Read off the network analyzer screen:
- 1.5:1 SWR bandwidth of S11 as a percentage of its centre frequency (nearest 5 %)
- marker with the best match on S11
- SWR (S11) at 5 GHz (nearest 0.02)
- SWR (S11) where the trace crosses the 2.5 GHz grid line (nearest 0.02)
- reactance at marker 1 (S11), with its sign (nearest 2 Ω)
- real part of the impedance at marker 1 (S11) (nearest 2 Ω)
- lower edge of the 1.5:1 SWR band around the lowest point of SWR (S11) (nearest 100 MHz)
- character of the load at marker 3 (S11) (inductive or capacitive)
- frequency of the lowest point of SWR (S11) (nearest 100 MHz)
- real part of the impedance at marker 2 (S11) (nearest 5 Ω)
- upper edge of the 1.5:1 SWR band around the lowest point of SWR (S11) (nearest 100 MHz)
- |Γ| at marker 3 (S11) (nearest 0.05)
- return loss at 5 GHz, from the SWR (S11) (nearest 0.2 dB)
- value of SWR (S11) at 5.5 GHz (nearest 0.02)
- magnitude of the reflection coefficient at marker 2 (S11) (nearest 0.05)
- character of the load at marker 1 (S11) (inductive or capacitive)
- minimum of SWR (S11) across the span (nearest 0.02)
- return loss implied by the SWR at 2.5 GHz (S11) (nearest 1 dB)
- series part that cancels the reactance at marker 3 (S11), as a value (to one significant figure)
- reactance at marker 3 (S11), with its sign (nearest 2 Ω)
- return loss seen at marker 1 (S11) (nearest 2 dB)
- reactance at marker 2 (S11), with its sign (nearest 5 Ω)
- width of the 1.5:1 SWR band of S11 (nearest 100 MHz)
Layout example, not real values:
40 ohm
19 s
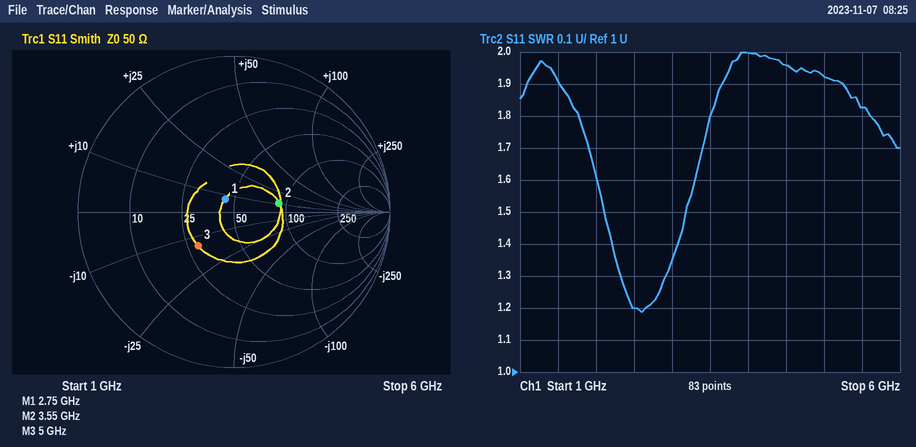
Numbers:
40 %
marker 1
1.92
1.20
+8 Ω
44 Ω
2.1 GHz
capacitive
2.6 GHz
90 Ω
3.2 GHz
0.30
10.0 dB
1.82
0.30
inductive
1.18
21 dB
400 pH
-14 Ω
20 dB
+10 Ω
1.1 GHz
